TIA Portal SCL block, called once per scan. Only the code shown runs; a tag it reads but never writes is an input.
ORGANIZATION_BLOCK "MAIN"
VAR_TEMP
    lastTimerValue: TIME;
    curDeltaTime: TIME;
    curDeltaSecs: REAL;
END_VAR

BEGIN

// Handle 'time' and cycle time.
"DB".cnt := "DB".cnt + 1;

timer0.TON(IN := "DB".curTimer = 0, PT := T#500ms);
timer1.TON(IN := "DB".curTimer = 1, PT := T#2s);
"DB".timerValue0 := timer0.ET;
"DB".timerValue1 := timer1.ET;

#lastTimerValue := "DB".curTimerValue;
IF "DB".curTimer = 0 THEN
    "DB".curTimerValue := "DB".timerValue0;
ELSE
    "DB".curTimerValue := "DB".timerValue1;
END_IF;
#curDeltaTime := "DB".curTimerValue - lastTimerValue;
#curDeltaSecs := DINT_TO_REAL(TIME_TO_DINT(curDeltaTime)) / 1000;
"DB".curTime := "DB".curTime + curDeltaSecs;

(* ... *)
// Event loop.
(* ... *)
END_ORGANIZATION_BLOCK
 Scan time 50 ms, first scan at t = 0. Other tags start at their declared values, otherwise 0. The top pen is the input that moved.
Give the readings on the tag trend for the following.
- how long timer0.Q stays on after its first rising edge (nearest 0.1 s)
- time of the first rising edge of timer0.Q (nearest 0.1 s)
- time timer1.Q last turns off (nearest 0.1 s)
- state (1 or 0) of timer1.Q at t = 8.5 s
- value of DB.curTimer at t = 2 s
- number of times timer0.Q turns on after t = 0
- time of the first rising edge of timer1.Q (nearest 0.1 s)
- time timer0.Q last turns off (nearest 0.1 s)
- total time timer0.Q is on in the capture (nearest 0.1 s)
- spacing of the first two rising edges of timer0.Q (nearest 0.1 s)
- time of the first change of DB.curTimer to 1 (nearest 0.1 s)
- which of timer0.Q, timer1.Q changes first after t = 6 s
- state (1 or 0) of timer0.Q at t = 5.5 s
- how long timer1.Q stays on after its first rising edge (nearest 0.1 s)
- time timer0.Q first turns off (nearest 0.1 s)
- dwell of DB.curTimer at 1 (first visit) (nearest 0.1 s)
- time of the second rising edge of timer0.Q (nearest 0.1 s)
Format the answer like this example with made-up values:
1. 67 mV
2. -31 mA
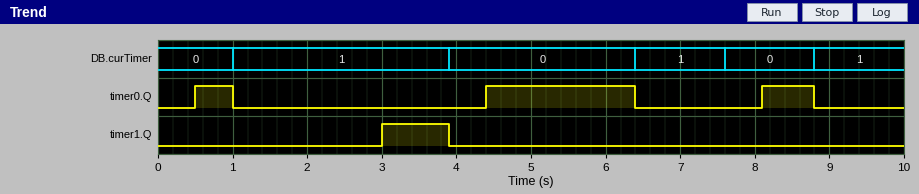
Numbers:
1. 0.5 s
2. 0.5 s
3. 3.9 s
4. 0
5. 1
6. 3
7. 3.0 s
8. 8.8 s
9. 3.2 s
10. 3.9 s
11. 1.0 s
12. timer0.Q
13. 1
14. 0.9 s
15. 1.0 s
16. 2.9 s
17. 4.4 s
